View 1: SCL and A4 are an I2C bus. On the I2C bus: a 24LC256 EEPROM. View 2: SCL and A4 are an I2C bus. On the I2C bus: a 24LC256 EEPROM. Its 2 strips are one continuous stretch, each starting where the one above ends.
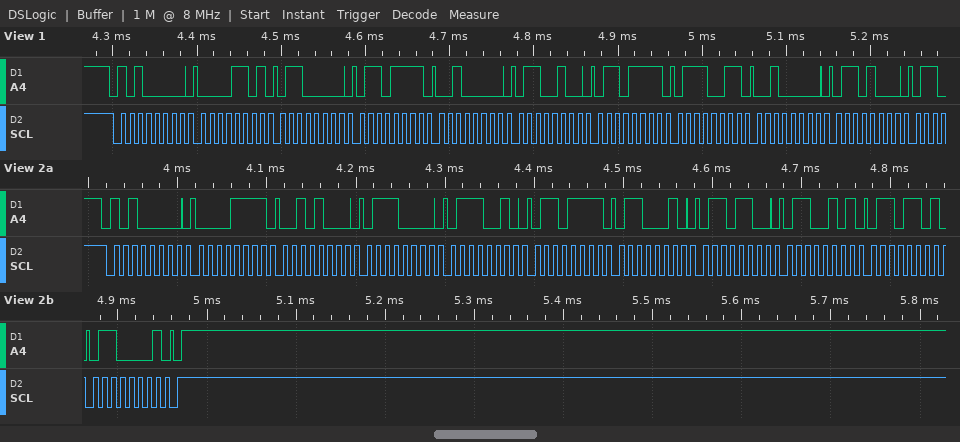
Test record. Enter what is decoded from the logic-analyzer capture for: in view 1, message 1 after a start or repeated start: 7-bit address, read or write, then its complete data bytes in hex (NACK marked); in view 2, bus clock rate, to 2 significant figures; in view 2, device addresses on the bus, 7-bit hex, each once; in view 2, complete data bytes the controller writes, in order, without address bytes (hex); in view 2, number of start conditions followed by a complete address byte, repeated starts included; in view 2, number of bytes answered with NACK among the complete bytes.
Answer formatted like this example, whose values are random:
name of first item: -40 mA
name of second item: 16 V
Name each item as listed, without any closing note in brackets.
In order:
in view 1, message 1 after a start or repeated start: 7-bit address, read or write, then its complete data bytes in hex: 0x50 write: 0D 60 6F 20 64 6F 73 20 68
in view 2, bus clock rate, to 2 significant figures: 100 kHz
in view 2, device addresses on the bus, 7-bit hex, each once: 0x50
in view 2, complete data bytes the controller writes, in order, without address bytes: 0F 28 70 72 6F 62 6C 65 6D 61
in view 2, number of start conditions followed by a complete address byte, repeated starts included: 1
in view 2, number of bytes answered with NACK among the complete bytes: 0
